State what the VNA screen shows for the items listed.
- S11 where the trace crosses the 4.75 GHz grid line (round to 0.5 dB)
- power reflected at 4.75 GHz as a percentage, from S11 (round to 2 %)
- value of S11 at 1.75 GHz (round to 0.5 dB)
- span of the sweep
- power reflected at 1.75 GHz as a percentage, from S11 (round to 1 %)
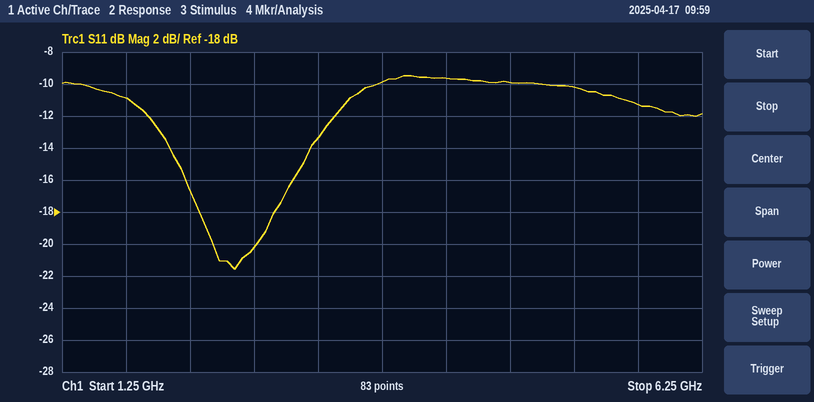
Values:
-10.0 dB
10 %
-11.0 dB
5 GHz
8 %
